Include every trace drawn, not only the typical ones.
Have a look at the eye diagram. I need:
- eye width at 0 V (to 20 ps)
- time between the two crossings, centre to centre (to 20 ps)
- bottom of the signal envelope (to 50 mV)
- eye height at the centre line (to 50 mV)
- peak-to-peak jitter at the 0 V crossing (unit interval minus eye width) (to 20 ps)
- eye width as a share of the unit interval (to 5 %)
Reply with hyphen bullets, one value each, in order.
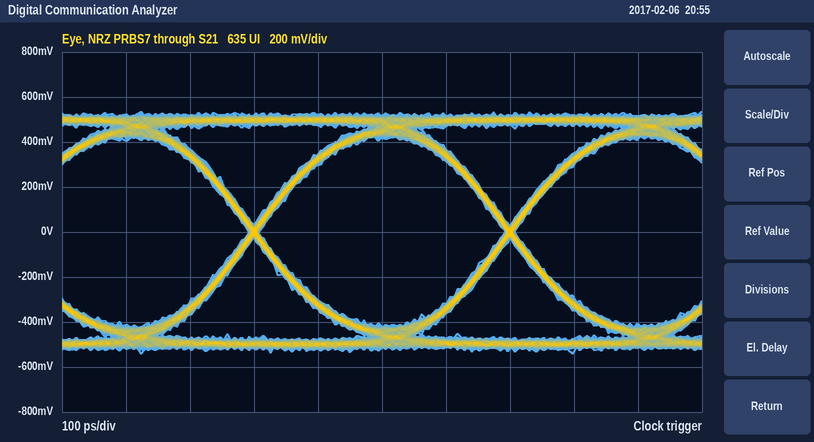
- 380 ps
- 400 ps
- -550 mV
- 850 mV
- 20 ps
- 95 %
